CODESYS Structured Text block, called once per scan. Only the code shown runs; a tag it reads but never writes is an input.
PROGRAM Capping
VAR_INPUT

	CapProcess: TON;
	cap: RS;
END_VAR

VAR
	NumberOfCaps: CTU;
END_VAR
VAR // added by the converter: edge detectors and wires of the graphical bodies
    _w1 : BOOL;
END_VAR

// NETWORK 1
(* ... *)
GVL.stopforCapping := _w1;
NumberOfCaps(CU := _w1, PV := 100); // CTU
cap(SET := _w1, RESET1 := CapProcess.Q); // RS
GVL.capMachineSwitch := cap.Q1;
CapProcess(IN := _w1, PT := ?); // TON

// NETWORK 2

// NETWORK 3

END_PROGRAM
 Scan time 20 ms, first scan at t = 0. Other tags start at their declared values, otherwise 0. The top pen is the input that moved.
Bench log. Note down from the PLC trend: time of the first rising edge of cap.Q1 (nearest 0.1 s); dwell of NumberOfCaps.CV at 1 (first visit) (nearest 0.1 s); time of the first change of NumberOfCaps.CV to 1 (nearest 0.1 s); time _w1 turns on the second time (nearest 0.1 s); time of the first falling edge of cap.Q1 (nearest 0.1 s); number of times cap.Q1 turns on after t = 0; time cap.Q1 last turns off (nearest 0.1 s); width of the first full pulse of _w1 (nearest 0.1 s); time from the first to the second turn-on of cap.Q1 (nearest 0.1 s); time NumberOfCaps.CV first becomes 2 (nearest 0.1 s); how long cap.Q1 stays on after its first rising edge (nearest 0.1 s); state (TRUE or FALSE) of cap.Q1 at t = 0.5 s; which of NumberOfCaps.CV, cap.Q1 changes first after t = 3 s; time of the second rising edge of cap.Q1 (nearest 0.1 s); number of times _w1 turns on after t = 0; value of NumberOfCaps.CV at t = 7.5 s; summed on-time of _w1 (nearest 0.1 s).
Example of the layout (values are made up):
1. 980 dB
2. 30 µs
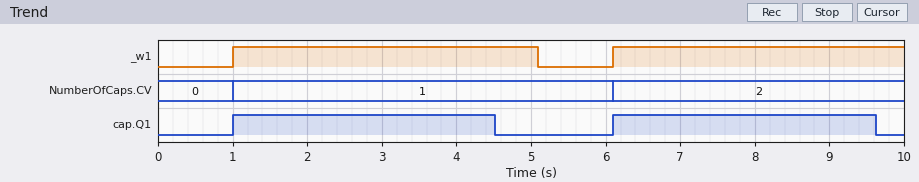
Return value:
1. 1.0 s
2. 5.1 s
3. 1.0 s
4. 6.1 s
5. 4.5 s
6. 2
7. 9.6 s
8. 4.1 s
9. 5.1 s
10. 6.1 s
11. 3.5 s
12. FALSE
13. cap.Q1
14. 6.1 s
15. 2
16. 2
17. 8.0 s
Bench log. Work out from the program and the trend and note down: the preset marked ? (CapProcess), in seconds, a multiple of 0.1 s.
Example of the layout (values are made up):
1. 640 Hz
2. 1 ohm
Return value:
1. 3.5 s
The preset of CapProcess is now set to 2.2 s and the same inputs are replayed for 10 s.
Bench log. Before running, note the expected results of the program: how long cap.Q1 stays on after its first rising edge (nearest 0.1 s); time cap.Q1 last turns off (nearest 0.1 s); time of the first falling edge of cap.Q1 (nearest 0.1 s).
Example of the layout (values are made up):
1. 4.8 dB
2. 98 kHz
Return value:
1. 2.2 s
2. 8.3 s
3. 3.2 s
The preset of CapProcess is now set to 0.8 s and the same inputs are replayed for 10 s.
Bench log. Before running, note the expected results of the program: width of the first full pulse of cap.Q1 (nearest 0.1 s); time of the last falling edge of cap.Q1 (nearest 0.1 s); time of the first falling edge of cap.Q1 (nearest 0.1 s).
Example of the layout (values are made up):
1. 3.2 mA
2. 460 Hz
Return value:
1. 0.8 s
2. 6.9 s
3. 1.8 s
